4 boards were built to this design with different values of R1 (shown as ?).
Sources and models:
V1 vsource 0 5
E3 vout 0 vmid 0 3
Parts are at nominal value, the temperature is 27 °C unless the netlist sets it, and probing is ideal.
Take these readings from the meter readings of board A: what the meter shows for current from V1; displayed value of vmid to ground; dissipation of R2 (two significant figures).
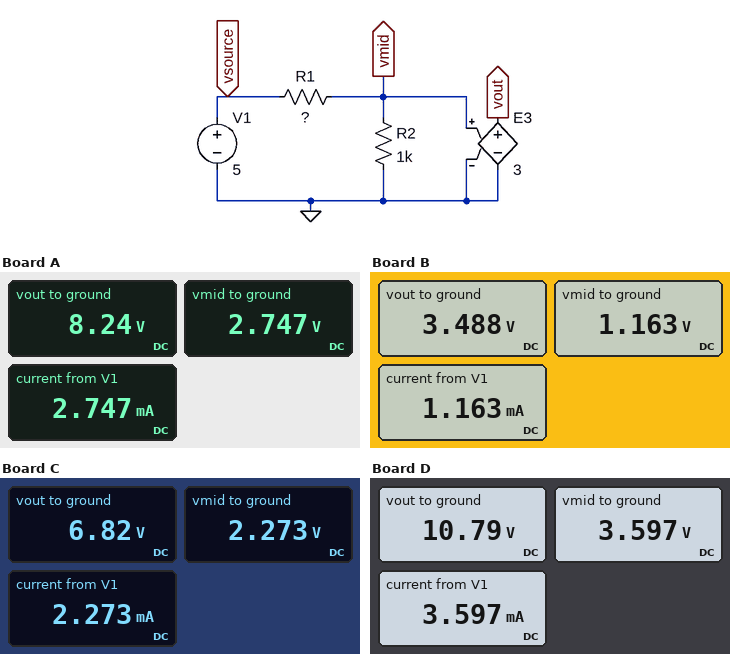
2.747 mA
2.747 V
7.5 mW
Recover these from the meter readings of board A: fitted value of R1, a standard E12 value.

820 Ω
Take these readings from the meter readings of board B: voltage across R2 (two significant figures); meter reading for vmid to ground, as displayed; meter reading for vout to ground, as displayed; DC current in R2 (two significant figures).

1.2 V
1.163 V
3.488 V
1.2 mA
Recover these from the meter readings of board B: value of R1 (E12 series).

3.3 kΩ
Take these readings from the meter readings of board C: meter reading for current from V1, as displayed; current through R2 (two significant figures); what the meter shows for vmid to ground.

2.273 mA
2.3 mA
2.273 V
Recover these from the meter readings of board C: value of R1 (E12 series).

1.2 kΩ
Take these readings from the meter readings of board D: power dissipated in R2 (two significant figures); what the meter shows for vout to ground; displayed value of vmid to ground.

13 mW
10.79 V
3.597 V
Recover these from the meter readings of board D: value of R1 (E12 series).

390 Ω
